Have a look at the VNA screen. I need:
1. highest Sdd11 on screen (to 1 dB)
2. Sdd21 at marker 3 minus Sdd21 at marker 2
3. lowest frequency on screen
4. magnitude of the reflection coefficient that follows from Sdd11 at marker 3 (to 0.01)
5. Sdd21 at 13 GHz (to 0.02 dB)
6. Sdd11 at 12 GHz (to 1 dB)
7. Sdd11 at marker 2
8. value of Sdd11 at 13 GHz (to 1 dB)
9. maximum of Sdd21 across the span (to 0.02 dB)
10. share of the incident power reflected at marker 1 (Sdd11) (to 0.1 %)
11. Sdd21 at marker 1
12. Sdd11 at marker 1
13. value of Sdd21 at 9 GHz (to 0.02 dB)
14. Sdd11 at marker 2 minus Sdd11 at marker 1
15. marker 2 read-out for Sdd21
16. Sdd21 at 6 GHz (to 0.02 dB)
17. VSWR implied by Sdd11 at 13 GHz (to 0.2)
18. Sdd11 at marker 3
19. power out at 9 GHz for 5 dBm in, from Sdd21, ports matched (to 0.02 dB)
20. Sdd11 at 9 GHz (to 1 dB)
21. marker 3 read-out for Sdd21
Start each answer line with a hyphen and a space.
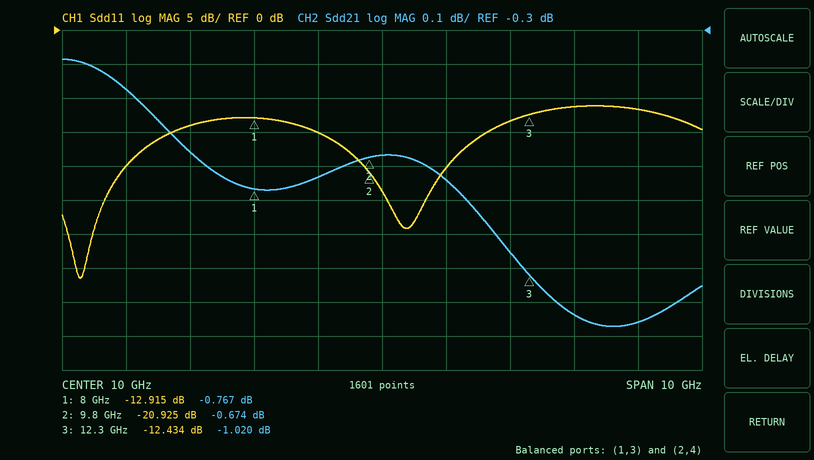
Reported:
- -11 dB
- -0.346 dB
- 5 GHz
- 0.24
- -1.14 dB
- -13 dB
- -20.925 dB
- -11 dB
- -0.38 dB
- 5.1 %
- -0.767 dB
- -12.915 dB
- -0.74 dB
- -8.010 dB
- -0.674 dB
- -0.48 dB
- 1.8
- -12.434 dB
- 4.26 dBm
- -15 dB
- -1.020 dB
